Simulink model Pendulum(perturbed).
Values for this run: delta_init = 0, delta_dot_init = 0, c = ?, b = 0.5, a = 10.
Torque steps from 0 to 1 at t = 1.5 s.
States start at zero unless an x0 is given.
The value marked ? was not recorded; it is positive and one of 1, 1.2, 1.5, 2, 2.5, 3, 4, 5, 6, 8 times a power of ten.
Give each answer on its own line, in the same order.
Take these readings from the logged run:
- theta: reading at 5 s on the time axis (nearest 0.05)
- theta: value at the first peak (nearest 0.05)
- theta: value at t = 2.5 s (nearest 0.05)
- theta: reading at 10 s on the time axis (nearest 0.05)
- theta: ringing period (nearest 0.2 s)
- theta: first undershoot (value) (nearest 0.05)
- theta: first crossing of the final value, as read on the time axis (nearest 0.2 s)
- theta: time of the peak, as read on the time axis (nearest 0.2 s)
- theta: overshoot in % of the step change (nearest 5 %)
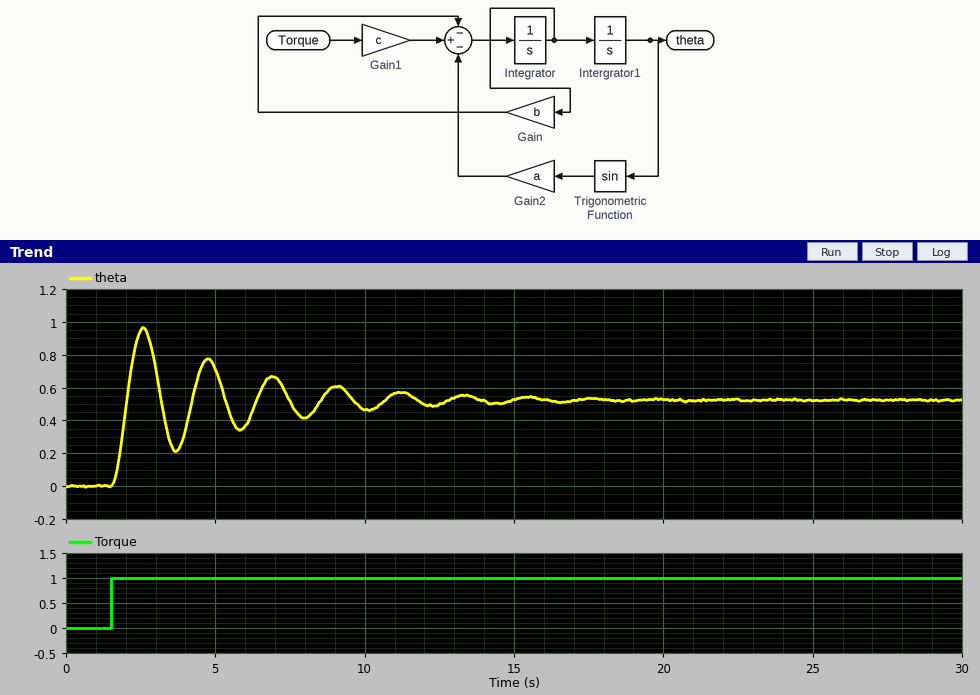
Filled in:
0.70
0.95
0.95
0.45
2.2 s
0.20
2.0 s
2.6 s
85 %
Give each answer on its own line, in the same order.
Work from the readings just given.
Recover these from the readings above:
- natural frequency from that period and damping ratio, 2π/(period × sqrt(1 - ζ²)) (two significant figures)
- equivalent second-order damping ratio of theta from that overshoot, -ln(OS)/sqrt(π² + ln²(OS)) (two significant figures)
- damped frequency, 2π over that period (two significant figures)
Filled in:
2.9 rad/s
0.052
2.9 rad/s
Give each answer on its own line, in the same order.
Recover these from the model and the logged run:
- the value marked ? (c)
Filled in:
5
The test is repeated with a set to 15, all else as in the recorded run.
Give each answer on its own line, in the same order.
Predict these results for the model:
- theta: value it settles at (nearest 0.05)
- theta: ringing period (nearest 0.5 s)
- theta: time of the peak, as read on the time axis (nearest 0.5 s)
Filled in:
0.35
1.5 s
2.5 s
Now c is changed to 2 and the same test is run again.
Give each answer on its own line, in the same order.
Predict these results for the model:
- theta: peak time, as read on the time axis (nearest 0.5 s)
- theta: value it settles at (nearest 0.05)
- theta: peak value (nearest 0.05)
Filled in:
2.5 s
0.20
0.35
